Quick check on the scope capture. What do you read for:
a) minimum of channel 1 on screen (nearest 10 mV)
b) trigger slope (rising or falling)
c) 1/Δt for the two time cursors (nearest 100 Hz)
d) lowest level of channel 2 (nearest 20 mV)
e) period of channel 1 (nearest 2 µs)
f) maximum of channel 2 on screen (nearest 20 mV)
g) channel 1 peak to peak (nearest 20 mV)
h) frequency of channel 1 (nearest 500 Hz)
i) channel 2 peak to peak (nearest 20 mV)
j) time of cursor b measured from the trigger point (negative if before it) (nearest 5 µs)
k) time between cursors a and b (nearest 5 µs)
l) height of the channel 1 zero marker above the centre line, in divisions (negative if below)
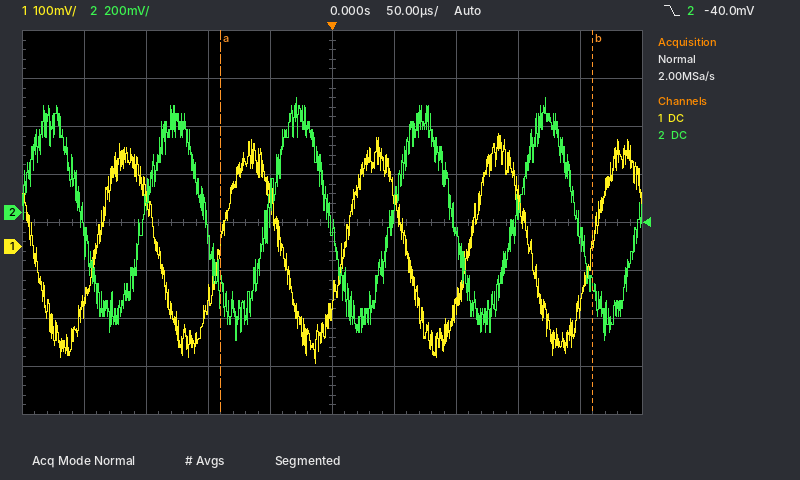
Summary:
-240 mV
falling
3.3 kHz
-540 mV
100 µs
480 mV
480 mV
10.0 kHz
1.02 V
+210 µs
300 µs
-0.5 div
